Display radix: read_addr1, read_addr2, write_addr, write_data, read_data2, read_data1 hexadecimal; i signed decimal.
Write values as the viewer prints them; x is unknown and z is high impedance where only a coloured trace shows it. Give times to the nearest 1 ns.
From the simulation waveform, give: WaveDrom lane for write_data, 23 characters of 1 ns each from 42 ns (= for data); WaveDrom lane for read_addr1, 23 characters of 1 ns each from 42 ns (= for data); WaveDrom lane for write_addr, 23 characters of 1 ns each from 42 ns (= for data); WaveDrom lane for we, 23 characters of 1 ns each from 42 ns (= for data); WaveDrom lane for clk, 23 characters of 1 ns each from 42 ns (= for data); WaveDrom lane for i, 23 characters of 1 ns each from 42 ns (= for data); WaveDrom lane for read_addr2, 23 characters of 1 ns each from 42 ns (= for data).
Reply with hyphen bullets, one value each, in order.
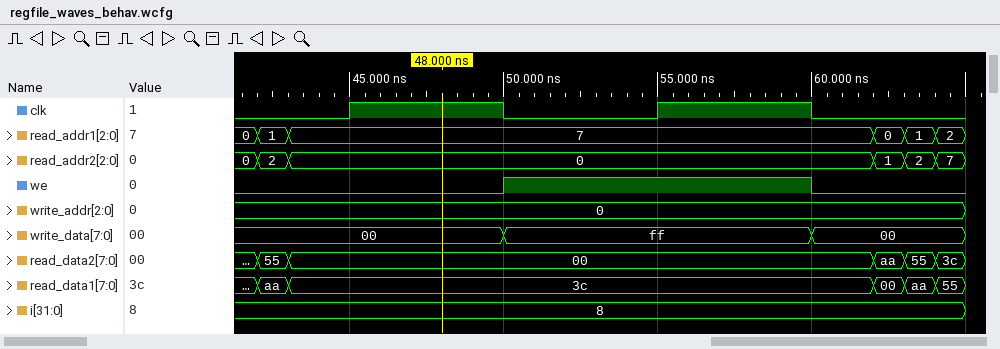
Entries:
- {name: 'write_data', wave: '=.......=.........=....', data: '00 ff 00'}
- {name: 'read_addr1', wave: '==..................===', data: '1 7 0 1 2'}
- {name: 'write_addr', wave: '=......................', data: '0'}
- {name: 'we', wave: '0.......1.........0....'}
- {name: 'clk', wave: '0..1....0....1....0....'}
- {name: 'i', wave: '=......................', data: '8'}
- {name: 'read_addr2', wave: '==..................===', data: '2 0 1 2 7'}
